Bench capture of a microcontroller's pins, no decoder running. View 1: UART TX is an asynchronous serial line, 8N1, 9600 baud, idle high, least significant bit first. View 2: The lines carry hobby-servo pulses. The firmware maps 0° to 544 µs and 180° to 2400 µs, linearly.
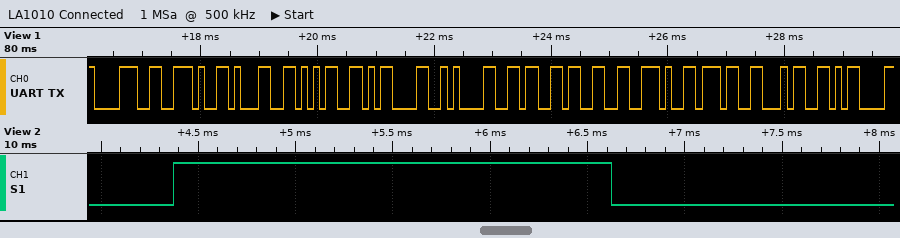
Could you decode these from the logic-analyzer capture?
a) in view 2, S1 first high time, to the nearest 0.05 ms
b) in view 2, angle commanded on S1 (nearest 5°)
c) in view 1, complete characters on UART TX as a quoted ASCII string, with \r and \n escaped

2.25 ms
165°
"8.15\r\n63.74\r"
